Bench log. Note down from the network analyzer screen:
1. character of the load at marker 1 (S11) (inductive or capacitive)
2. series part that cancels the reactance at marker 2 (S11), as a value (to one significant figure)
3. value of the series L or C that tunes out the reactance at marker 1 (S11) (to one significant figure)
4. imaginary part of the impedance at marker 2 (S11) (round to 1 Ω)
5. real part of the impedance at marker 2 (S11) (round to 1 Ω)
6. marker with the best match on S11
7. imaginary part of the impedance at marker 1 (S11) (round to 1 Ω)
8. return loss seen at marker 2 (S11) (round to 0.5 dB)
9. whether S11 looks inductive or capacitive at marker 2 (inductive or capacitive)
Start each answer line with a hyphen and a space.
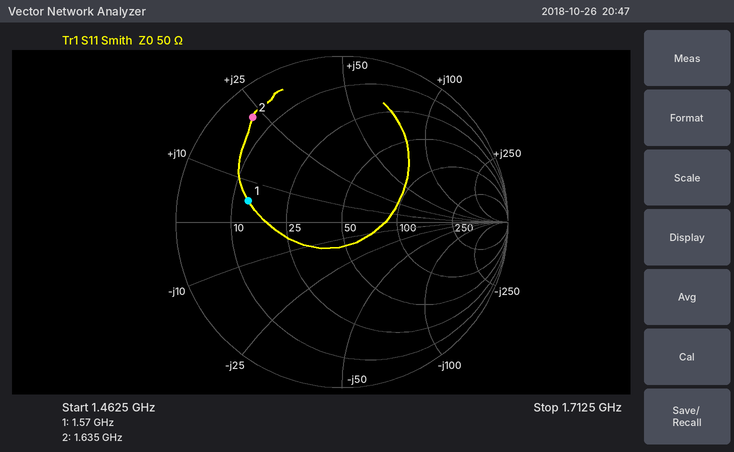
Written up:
- inductive
- 4 pF
- 20 pF
- +23 Ω
- 6 Ω
- marker 1
- +5 Ω
- 1.5 dB
- inductive
